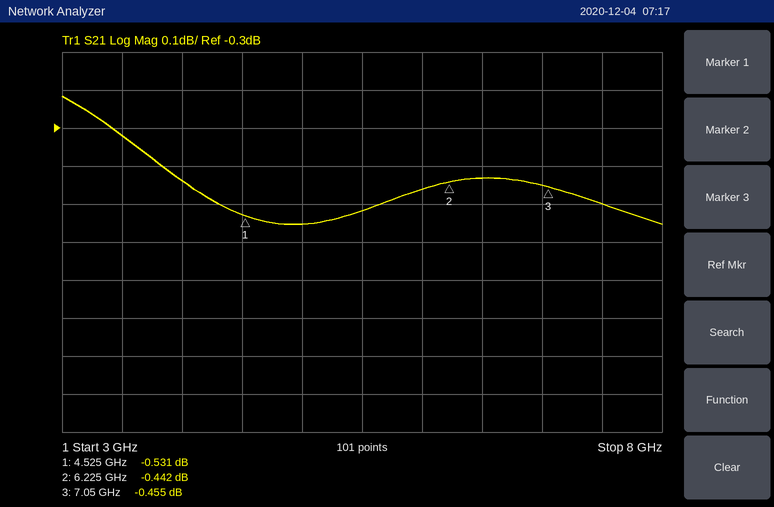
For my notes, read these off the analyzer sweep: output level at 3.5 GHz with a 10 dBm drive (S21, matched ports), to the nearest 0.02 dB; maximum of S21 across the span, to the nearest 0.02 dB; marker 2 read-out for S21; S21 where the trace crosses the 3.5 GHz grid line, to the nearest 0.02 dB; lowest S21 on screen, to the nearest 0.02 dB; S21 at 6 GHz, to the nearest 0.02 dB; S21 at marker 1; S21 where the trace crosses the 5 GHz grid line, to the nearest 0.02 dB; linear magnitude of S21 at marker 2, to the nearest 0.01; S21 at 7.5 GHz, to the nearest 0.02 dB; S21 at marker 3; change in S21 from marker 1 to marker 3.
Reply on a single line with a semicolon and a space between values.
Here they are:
9.68 dBm; -0.22 dB; -0.442 dB; -0.32 dB; -0.56 dB; -0.46 dB; -0.531 dB; -0.56 dB; 0.95; -0.50 dB; -0.455 dB; 0.076 dB
